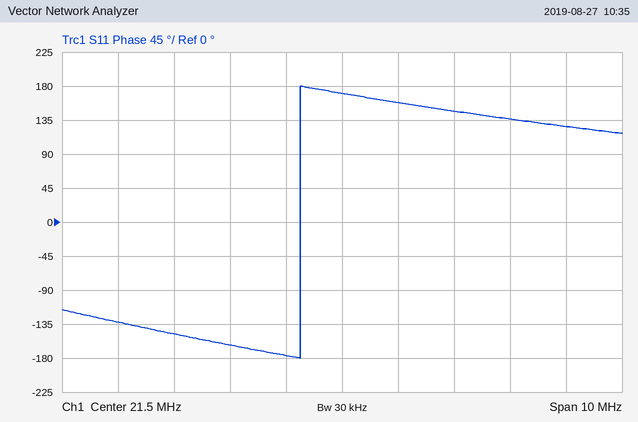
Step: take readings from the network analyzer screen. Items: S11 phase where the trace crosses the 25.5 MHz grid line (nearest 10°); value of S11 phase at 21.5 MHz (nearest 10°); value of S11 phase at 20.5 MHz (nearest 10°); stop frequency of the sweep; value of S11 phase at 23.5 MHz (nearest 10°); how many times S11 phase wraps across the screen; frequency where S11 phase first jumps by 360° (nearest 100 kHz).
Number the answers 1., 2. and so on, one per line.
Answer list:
1. 130°
2. 170°
3. -180°
4. 26.5 MHz
5. 150°
6. 1
7. 20.8 MHz
